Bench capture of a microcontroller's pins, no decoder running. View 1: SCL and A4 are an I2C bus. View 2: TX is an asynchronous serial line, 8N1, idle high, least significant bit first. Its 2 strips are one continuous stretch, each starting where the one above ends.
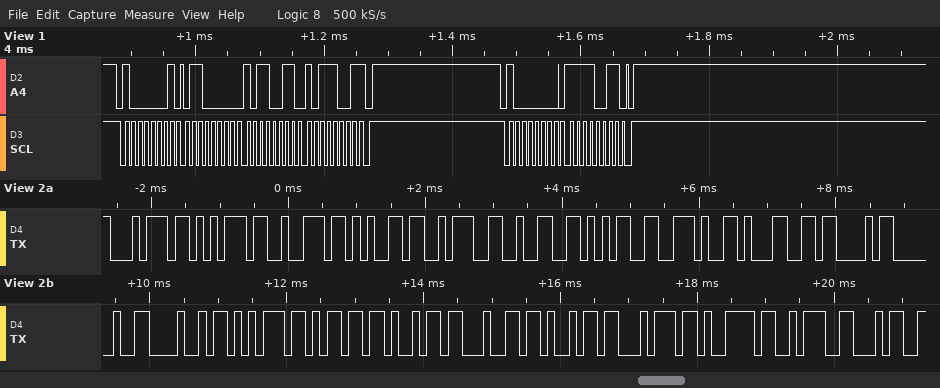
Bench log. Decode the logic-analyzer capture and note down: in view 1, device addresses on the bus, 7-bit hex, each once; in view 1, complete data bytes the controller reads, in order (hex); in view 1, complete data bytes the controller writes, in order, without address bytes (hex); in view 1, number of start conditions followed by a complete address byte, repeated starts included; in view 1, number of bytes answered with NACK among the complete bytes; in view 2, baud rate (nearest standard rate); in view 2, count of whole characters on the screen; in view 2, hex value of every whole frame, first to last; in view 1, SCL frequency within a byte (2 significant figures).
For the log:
0x40
60 B3 B9
F3
2
1
9600 baud
21
74 75 72 65 3A 32 35 2E 31 43 20 48 75 6D 69 64 69 74 79 3A 34
100 kHz
